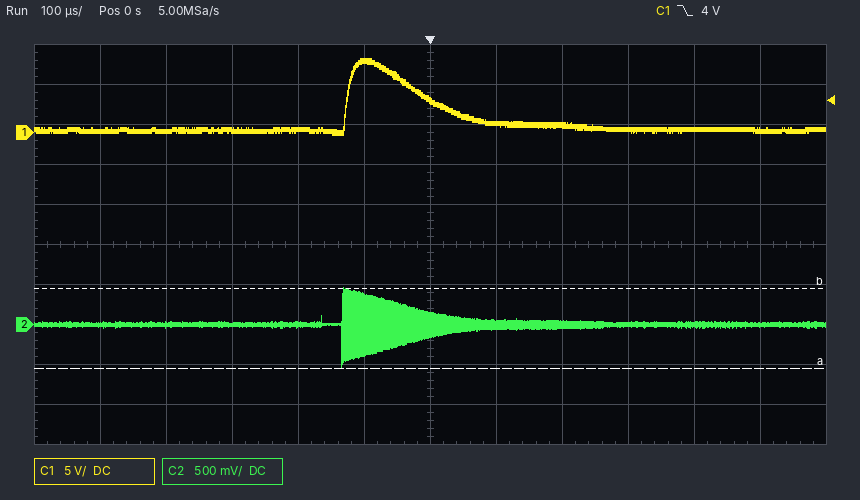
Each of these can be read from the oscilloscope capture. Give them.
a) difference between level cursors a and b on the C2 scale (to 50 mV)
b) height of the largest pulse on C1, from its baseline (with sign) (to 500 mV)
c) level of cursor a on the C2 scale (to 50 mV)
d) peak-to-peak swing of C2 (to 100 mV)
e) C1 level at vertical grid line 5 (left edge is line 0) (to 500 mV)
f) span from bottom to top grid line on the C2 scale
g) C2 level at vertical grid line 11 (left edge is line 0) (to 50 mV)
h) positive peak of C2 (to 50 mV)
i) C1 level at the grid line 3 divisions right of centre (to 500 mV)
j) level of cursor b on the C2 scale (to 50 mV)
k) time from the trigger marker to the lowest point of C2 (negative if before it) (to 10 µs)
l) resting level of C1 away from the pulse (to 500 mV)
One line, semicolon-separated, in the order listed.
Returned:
1.00 V; +9.0 V; -550 mV; 1.00 V; 9.0 V; 5 V; 0 mV; 450 mV; 500 mV; 450 mV; -130 µs; 500 mV
